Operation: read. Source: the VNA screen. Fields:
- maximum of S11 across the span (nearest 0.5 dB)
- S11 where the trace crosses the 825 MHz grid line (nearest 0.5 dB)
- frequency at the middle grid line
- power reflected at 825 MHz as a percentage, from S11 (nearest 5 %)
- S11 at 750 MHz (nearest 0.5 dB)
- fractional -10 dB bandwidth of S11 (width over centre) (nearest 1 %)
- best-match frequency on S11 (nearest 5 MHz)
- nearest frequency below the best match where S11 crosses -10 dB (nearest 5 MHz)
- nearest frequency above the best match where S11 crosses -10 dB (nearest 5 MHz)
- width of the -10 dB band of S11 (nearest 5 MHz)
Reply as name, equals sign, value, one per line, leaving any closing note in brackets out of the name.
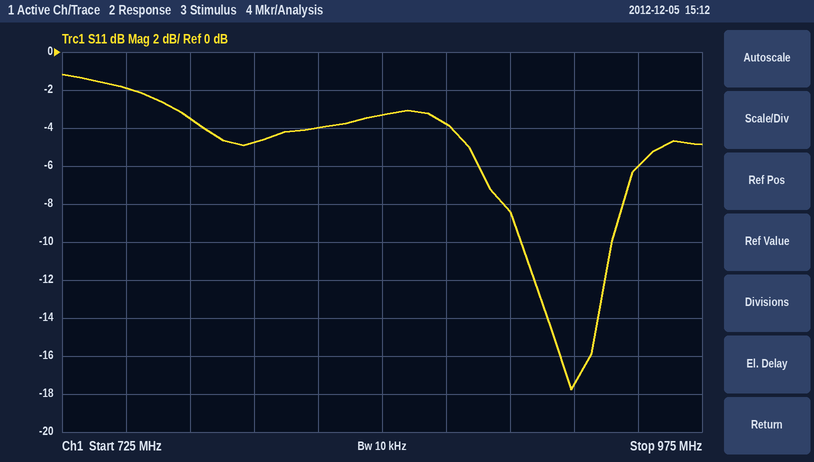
maximum of S11 across the span = -1.0 dB
S11 where the trace crosses the 825 MHz grid line = -4.0 dB
frequency at the middle grid line = 850 MHz
power reflected at 825 MHz as a percentage, from S11 = 40 %
S11 at 750 MHz = -2.0 dB
fractional -10 dB bandwidth of S11 (width over centre) = 4 %
best-match frequency on S11 = 925 MHz
nearest frequency below the best match where S11 crosses -10 dB = 905 MHz
nearest frequency above the best match where S11 crosses -10 dB = 940 MHz
width of the -10 dB band of S11 = 35 MHz
